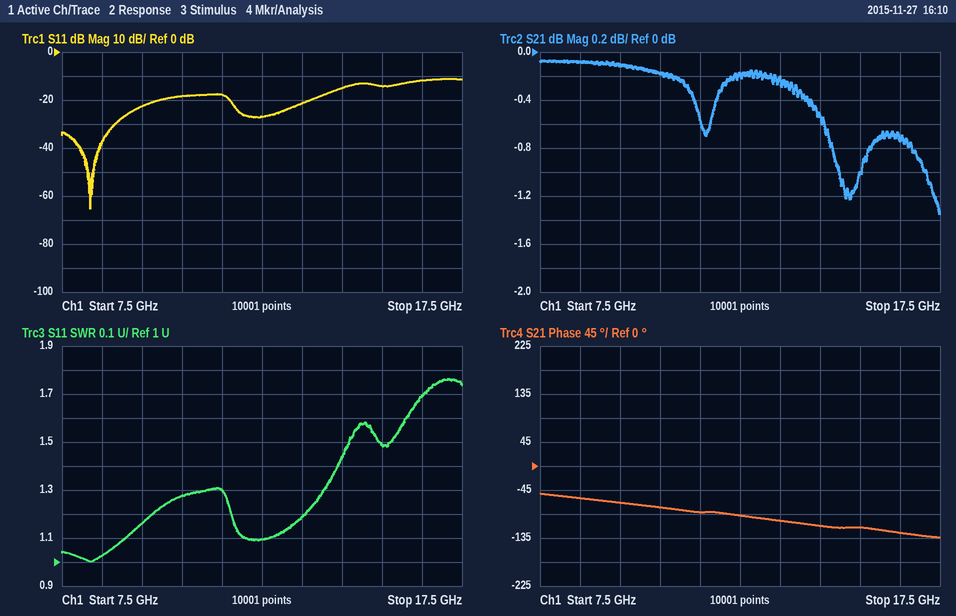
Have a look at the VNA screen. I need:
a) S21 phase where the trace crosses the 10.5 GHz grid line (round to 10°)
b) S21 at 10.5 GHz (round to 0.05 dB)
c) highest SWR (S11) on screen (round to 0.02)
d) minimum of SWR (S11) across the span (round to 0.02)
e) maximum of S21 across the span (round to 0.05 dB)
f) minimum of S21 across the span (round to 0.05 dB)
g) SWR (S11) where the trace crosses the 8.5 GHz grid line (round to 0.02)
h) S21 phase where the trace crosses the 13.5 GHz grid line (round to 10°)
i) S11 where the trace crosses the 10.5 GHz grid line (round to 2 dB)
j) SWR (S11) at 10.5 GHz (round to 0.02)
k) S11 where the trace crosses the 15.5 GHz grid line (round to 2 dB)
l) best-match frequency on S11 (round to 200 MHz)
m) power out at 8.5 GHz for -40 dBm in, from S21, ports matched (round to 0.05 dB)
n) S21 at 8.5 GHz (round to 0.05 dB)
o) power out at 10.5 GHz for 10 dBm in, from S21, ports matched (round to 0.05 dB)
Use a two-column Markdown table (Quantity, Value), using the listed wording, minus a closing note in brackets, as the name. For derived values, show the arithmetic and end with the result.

| Quantity | Value |
|---|---|
| S21 phase where the trace crosses the 10.5 GHz grid line | -80° |
| S21 at 10.5 GHz | -0.20 dB |
| highest SWR (S11) on screen | 1.76 |
| minimum of SWR (S11) across the span | 1.00 |
| maximum of S21 across the span | -0.05 dB |
| minimum of S21 across the span | -1.35 dB |
| SWR (S11) where the trace crosses the 8.5 GHz grid line | 1.02 |
| S21 phase where the trace crosses the 13.5 GHz grid line | -100° |
| S11 where the trace crosses the 10.5 GHz grid line | -18 dB |
| SWR (S11) at 10.5 GHz | 1.28 |
| S11 where the trace crosses the 15.5 GHz grid line | -14 dB |
| best-match frequency on S11 | 8.2 GHz |
| power out at 8.5 GHz for -40 dBm in, from S21, ports matched | -40 dBm + (-0.10 dB) = -40.10 dBm |
| S21 at 8.5 GHz | -0.10 dB |
| power out at 10.5 GHz for 10 dBm in, from S21, ports matched | 10 dBm + (-0.20 dB) = 9.80 dBm |
